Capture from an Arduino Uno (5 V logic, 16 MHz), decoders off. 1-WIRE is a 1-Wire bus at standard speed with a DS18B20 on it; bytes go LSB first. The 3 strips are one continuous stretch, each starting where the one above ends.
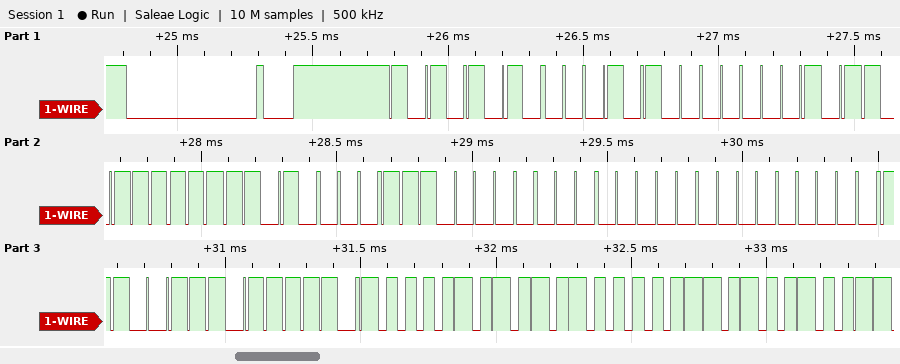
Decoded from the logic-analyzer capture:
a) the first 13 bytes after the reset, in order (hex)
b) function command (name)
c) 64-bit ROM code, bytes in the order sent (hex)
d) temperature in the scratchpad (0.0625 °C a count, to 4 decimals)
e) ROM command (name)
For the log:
55 28 A0 FD 0B 07 00 00 E6 BE 50 05 4B
Read Scratchpad
28 A0 FD 0B 07 00 00 E6
85.0000 °C
Match ROM
